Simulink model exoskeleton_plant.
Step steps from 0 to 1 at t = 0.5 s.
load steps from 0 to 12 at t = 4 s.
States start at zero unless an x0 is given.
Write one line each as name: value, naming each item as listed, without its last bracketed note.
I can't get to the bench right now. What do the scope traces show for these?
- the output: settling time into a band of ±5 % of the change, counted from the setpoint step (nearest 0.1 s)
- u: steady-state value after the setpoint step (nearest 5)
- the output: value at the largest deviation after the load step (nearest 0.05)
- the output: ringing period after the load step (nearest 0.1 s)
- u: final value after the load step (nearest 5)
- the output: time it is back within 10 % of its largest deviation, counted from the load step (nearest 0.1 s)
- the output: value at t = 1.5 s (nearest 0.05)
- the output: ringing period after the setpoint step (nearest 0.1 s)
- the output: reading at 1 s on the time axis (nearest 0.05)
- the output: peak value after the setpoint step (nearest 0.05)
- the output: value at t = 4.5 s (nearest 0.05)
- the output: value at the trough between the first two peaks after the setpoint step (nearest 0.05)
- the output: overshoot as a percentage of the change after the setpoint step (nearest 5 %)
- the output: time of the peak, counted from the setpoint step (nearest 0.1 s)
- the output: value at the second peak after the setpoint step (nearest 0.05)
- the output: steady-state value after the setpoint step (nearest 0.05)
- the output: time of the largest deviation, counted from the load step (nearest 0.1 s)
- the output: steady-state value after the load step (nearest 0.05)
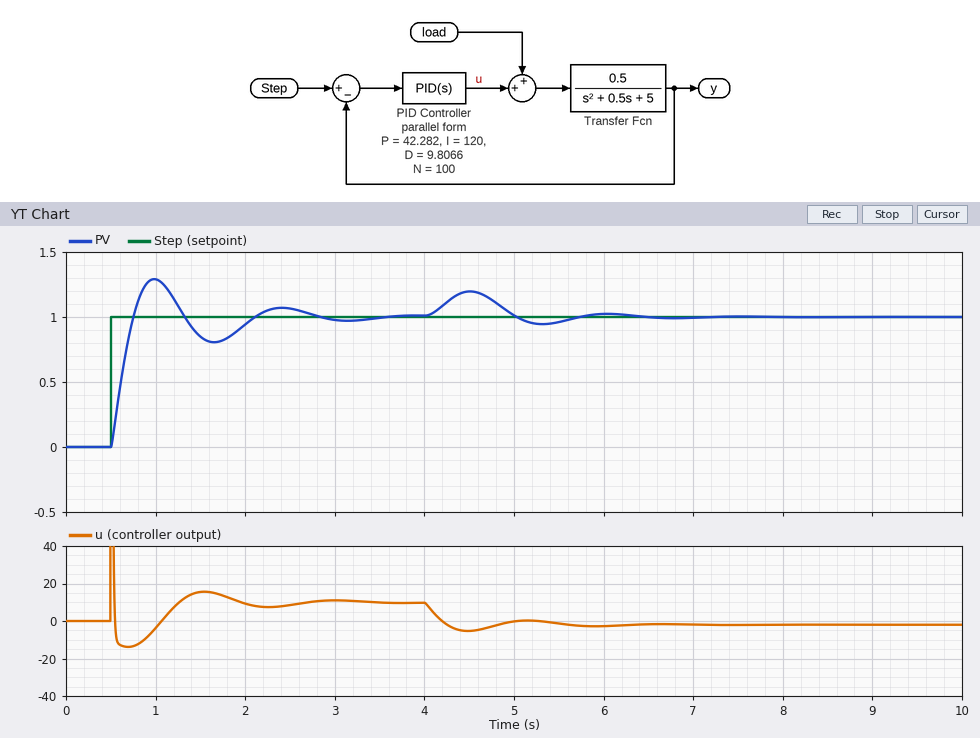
the output: settling time into a band of ±5 % of the change, counted from the setpoint step: 2.1 s
u: steady-state value after the setpoint step: 10
the output: value at the largest deviation after the load step: 1.20
the output: ringing period after the load step: 1.5 s
u: final value after the load step: 0
the output: time it is back within 10 % of its largest deviation, counted from the load step: 2.2 s
the output: value at t = 1.5 s: 0.85
the output: ringing period after the setpoint step: 1.4 s
the output: reading at 1 s on the time axis: 1.30
the output: peak value after the setpoint step: 1.30
the output: value at t = 4.5 s: 1.20
the output: value at the trough between the first two peaks after the setpoint step: 0.80
the output: overshoot as a percentage of the change after the setpoint step: 30 %
the output: time of the peak, counted from the setpoint step: 0.5 s
the output: value at the second peak after the setpoint step: 1.05
the output: steady-state value after the setpoint step: 1.00
the output: time of the largest deviation, counted from the load step: 0.5 s
the output: steady-state value after the load step: 1.00
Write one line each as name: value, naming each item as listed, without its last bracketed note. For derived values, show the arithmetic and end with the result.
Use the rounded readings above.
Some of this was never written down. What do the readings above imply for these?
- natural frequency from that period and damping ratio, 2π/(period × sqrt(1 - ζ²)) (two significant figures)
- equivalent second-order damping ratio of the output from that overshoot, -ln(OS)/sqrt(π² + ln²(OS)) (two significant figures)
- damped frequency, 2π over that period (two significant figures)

natural frequency from that period and damping ratio, 2π/(period × sqrt(1 - ζ²)): 2π / (1.4 × sqrt(1 - 0.36²)) = 4.8 rad/s
equivalent second-order damping ratio of the output from that overshoot, -ln(OS)/sqrt(π² + ln²(OS)): ln(0.3) = -1.204; 1.204 / sqrt(9.870 + 1.450) = 0.36
damped frequency, 2π over that period: 2π / 1.4 = 4.5 rad/s
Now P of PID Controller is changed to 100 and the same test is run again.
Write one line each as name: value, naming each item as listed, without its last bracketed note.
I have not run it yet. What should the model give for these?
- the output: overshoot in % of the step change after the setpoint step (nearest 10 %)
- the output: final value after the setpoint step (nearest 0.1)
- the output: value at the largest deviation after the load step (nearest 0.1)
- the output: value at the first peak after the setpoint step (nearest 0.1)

the output: overshoot in % of the step change after the setpoint step: 40 %
the output: final value after the setpoint step: 1.0
the output: value at the largest deviation after the load step: 1.1
the output: value at the first peak after the setpoint step: 1.4
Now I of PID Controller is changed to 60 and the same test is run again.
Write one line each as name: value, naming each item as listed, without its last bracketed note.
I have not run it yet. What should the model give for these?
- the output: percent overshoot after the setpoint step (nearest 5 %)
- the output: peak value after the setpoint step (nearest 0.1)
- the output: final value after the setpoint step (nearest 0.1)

the output: percent overshoot after the setpoint step: 20 %
the output: peak value after the setpoint step: 1.2
the output: final value after the setpoint step: 1.0
